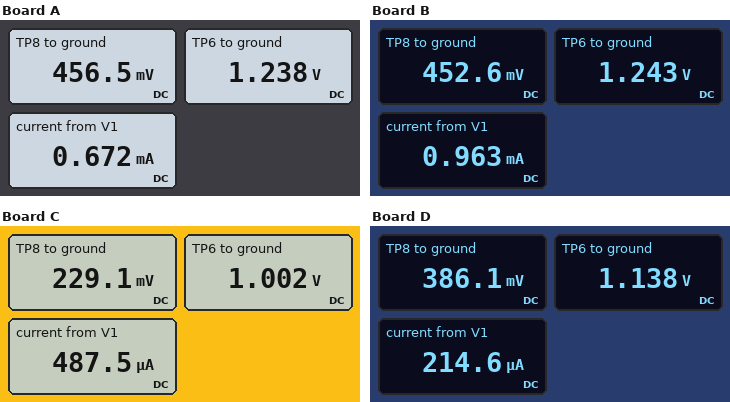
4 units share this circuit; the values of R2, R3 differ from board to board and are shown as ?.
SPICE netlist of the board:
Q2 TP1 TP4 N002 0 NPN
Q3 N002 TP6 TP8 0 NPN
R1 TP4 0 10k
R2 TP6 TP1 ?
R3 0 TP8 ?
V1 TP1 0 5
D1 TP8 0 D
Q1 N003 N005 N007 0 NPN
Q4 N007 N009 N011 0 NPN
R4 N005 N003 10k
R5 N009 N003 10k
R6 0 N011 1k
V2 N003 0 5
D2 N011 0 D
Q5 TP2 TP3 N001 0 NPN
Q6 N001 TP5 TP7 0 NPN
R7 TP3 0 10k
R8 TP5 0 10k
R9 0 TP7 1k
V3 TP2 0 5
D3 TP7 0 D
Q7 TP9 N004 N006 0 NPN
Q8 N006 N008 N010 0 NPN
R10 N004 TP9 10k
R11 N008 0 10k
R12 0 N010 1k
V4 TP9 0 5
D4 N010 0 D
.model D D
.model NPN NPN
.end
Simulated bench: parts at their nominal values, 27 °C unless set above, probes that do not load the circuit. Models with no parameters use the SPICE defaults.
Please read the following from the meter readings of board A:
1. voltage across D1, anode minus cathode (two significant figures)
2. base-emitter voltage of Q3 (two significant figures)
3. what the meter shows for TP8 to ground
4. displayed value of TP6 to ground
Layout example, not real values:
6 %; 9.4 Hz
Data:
460 mV; 780 mV; 456.5 mV; 1.238 V
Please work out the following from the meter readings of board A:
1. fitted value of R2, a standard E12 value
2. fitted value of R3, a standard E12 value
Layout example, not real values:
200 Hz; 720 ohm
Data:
5.6 kΩ; 680 Ω
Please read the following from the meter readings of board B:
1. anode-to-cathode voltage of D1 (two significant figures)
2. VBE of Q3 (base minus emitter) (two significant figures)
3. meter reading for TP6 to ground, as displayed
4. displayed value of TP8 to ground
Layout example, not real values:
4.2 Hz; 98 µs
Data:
450 mV; 790 mV; 1.243 V; 452.6 mV
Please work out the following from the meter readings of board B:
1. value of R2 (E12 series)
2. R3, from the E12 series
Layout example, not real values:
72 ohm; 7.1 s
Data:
3.9 kΩ; 470 Ω
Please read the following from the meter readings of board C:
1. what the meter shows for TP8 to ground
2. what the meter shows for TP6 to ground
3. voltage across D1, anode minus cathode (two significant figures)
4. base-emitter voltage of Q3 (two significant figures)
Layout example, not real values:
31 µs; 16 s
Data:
229.1 mV; 1.002 V; 230 mV; 770 mV
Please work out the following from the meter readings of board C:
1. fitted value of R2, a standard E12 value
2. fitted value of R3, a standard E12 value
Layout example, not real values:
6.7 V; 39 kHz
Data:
8.2 kΩ; 470 Ω
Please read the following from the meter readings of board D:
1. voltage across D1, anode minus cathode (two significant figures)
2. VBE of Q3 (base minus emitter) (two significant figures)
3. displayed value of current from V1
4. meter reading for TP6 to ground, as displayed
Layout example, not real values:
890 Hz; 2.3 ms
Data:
390 mV; 750 mV; 214.6 µA; 1.138 V
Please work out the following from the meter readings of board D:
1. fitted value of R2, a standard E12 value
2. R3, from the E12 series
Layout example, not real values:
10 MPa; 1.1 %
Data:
18 kΩ; 1.8 kΩ
